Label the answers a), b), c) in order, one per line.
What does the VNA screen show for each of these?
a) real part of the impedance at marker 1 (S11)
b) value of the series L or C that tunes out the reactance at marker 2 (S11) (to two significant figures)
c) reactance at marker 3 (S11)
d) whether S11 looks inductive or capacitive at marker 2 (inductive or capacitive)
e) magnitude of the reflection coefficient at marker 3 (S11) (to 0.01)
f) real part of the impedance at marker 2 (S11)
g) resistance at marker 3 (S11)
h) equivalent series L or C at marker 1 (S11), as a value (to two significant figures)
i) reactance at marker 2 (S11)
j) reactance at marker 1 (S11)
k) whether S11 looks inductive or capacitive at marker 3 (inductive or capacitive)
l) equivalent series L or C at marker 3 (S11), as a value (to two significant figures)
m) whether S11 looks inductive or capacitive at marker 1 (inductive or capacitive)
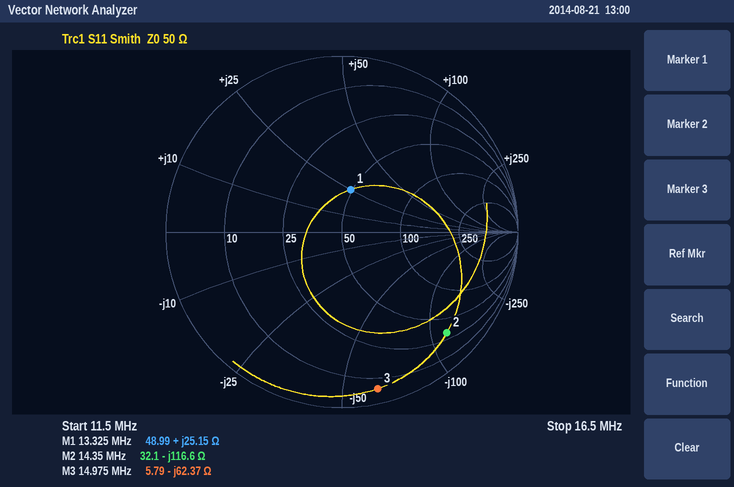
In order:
a) 48.99 Ω
b) 1.3 µH
c) -62.37 Ω
d) capacitive
e) 0.91
f) 32.1 Ω
g) 5.79 Ω
h) 300 nH
i) -116.6 Ω
j) +25.15 Ω
k) capacitive
l) 170 pF
m) inductive
